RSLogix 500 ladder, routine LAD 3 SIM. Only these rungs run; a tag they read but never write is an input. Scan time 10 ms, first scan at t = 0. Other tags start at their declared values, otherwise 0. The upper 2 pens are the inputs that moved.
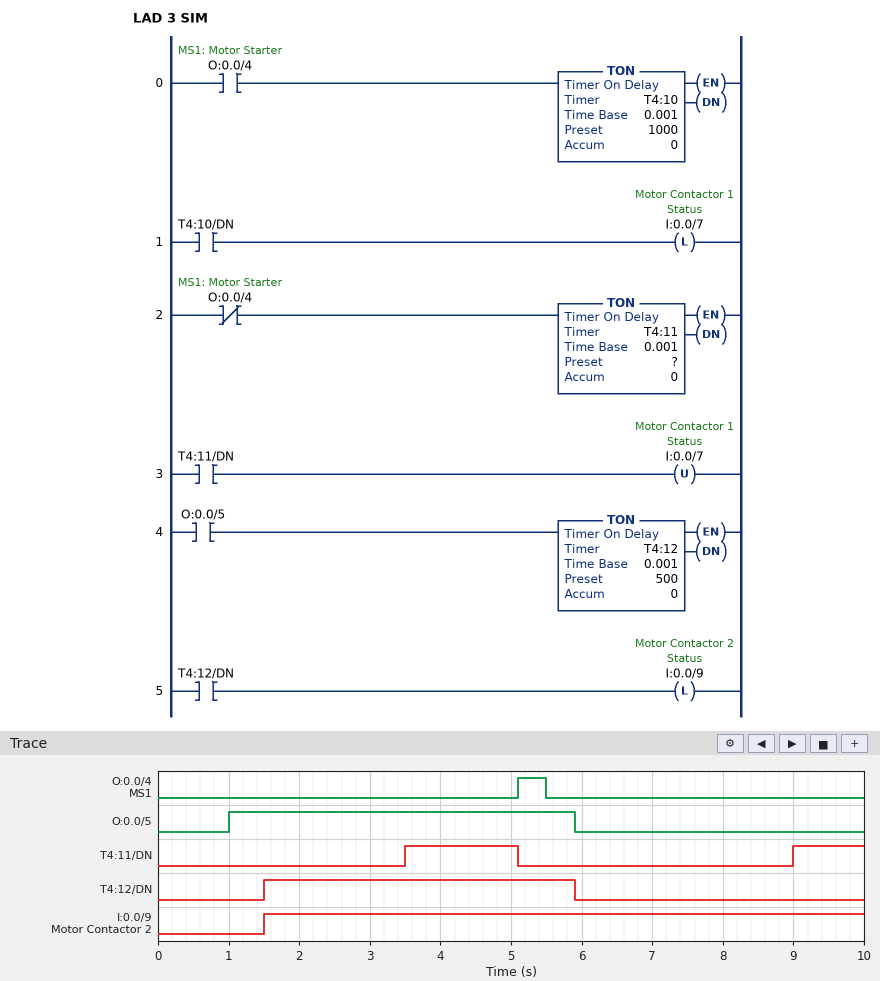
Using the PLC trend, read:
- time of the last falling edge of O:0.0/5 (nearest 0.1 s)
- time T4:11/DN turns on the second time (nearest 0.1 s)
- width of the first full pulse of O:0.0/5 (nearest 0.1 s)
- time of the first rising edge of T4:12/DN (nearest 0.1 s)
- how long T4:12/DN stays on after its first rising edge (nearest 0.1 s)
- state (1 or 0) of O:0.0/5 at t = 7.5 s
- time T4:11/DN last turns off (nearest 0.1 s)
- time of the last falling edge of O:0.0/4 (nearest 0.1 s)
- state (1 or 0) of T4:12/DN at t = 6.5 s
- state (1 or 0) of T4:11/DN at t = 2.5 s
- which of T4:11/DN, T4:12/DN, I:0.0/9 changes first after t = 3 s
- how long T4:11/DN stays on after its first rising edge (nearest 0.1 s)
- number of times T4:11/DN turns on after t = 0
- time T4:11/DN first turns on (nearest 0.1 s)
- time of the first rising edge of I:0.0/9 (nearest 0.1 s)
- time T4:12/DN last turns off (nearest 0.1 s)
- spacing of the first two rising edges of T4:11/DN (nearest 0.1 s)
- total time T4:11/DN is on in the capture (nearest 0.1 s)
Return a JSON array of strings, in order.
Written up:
["5.9 s", "9.0 s", "4.9 s", "1.5 s", "4.4 s", "0", "5.1 s", "5.5 s", "0", "0", "T4:11/DN", "1.6 s", "2", "3.5 s", "1.5 s", "5.9 s", "5.5 s", "2.6 s"]
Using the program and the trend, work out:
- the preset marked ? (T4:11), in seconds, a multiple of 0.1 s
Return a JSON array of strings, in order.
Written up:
["3.5 s"]
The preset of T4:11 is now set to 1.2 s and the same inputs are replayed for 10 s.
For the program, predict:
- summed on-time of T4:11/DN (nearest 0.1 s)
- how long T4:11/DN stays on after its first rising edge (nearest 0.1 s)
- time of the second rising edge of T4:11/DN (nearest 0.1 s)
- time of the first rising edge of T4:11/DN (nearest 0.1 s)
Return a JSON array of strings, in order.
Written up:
["7.2 s", "3.9 s", "6.7 s", "1.2 s"]
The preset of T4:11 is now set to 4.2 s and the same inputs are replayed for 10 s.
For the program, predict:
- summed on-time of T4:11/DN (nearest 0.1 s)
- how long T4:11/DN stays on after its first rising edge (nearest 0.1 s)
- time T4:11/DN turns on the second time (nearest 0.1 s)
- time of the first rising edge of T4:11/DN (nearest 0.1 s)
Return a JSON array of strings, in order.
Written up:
["1.2 s", "0.9 s", "9.7 s", "4.2 s"]
